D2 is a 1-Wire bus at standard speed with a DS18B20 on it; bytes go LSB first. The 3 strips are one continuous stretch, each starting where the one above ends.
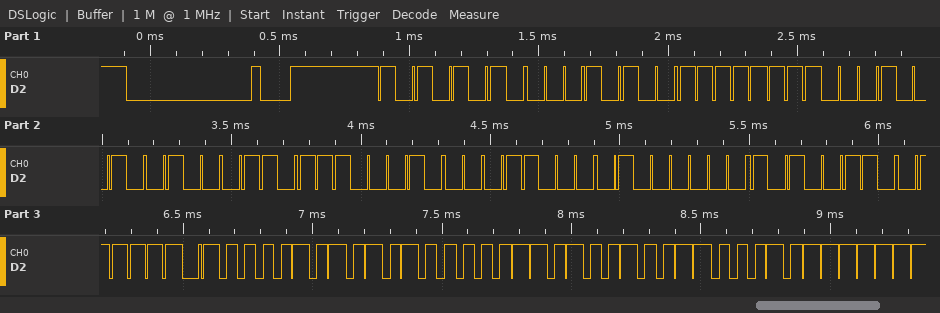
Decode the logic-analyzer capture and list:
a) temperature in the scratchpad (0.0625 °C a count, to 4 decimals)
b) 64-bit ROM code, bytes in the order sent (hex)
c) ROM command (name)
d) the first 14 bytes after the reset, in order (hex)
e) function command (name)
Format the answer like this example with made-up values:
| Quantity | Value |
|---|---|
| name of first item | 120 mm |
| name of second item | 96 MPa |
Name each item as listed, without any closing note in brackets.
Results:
| Quantity | Value |
|---|---|
| temperature in the scratchpad | 85.0000 °C |
| 64-bit ROM code, bytes in the order sent | 28 FF 48 62 47 18 02 65 |
| ROM command | Match ROM |
| the first 14 bytes after the reset, in order | 55 28 FF 48 62 47 18 02 65 BE 50 05 4B 46 |
| function command | Read Scratchpad |
